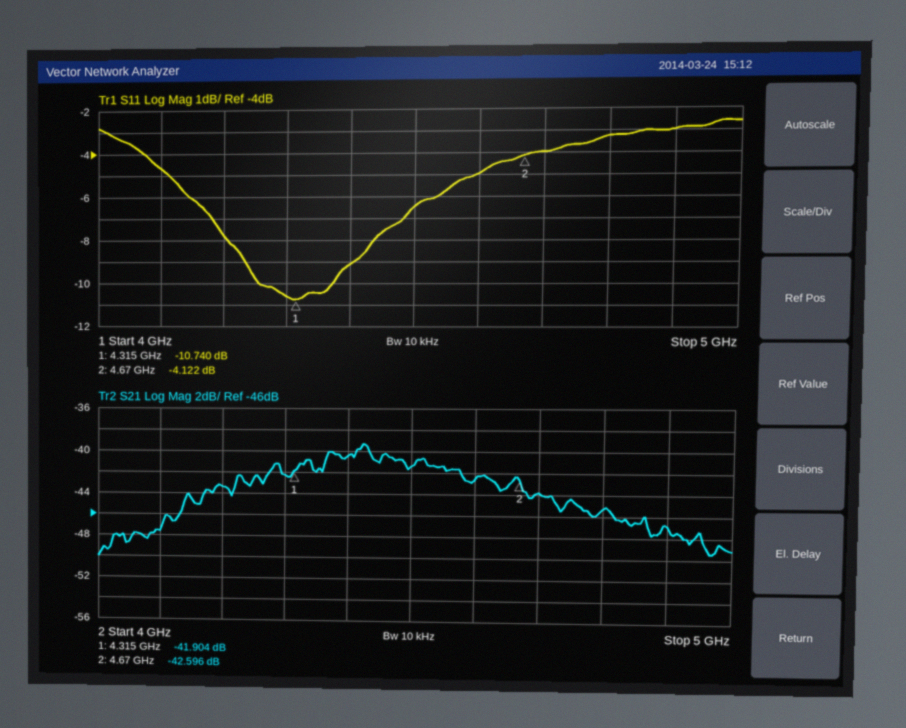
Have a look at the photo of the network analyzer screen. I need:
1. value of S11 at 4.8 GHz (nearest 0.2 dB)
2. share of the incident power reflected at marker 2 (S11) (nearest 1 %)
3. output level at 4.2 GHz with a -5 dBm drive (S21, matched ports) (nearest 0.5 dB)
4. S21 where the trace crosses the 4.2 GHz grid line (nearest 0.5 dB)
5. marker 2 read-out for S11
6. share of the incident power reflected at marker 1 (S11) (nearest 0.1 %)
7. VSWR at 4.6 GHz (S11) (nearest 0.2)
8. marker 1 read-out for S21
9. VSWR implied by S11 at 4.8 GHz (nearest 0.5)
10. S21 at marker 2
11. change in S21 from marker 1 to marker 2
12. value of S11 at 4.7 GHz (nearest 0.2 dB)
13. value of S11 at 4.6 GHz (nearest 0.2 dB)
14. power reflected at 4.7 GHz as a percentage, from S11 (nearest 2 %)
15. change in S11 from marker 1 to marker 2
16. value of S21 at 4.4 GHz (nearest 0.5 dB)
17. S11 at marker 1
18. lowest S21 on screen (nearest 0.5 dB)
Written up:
-3.2 dB
39 %
-48.5 dBm
-43.5 dB
-4.122 dB
8.4 %
3.6
-41.904 dB
5.5
-42.596 dB
-0.692 dB
-4.0 dB
-5.0 dB
40 %
6.618 dB
-40.5 dB
-10.740 dB
-50.0 dB
